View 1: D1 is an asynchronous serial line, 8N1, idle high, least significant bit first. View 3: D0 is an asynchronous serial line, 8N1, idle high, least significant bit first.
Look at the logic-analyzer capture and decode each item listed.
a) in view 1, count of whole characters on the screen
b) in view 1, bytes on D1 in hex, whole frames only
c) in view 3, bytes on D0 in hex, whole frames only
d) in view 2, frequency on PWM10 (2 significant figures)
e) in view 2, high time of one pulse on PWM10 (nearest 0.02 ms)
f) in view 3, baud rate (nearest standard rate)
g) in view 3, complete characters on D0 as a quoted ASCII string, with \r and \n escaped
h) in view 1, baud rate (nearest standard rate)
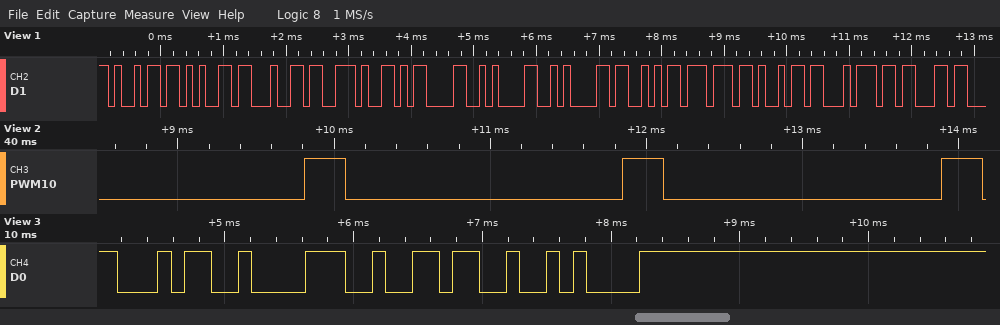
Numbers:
12
0x69 0x65 0x64 0x2E 0x0D 0x0A 0x0A 0x53 0x77 0x69 0x74 0x63
34 38 36 0A
490 Hz
0.26 ms
9600 baud
"486\n"
9600 baud
